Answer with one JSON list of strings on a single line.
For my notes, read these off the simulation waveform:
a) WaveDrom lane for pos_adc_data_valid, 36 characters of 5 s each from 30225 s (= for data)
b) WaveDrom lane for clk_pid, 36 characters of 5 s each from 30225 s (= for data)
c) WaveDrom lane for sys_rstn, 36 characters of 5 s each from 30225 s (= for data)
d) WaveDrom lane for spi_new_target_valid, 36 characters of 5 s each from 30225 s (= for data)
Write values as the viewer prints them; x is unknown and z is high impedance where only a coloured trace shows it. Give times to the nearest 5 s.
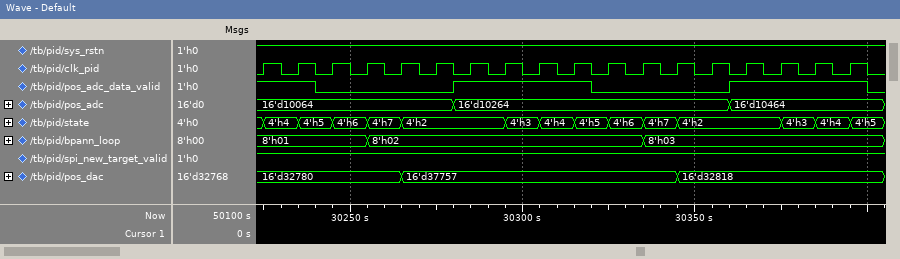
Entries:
["{name: 'pos_adc_data_valid', wave: '1..0.......1.......0.......1.......0'}", "{name: 'clk_pid', wave: '101010101010101010101010101010101010'}", "{name: 'sys_rstn', wave: '1...................................'}", "{name: 'spi_new_target_valid', wave: '1...................................'}"]
